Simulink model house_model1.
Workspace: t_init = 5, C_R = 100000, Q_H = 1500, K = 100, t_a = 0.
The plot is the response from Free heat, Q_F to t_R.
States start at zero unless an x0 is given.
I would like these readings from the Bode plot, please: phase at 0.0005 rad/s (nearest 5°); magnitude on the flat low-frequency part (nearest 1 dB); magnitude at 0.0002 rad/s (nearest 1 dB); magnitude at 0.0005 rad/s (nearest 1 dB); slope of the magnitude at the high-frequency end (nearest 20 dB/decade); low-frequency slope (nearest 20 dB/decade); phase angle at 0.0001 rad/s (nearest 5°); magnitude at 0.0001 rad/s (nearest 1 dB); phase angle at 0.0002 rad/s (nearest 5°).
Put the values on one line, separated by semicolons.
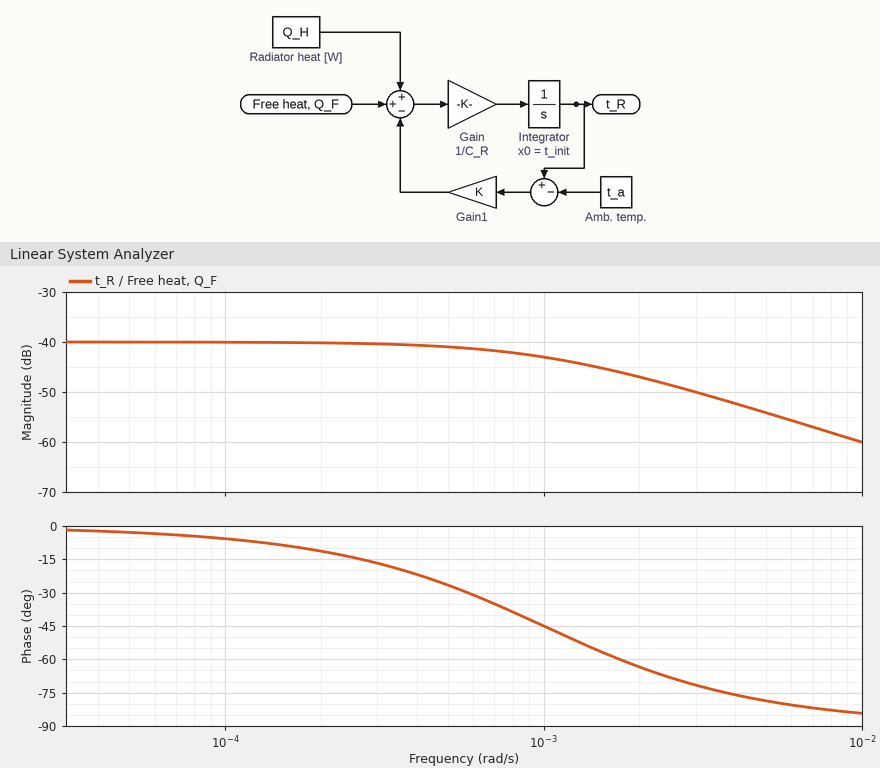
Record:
-25°; -40 dB; -40 dB; -41 dB; -20 dB/decade; 0 dB/decade; -5°; -40 dB; -10°
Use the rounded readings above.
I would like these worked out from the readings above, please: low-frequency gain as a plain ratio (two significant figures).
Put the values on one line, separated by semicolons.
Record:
0.010
